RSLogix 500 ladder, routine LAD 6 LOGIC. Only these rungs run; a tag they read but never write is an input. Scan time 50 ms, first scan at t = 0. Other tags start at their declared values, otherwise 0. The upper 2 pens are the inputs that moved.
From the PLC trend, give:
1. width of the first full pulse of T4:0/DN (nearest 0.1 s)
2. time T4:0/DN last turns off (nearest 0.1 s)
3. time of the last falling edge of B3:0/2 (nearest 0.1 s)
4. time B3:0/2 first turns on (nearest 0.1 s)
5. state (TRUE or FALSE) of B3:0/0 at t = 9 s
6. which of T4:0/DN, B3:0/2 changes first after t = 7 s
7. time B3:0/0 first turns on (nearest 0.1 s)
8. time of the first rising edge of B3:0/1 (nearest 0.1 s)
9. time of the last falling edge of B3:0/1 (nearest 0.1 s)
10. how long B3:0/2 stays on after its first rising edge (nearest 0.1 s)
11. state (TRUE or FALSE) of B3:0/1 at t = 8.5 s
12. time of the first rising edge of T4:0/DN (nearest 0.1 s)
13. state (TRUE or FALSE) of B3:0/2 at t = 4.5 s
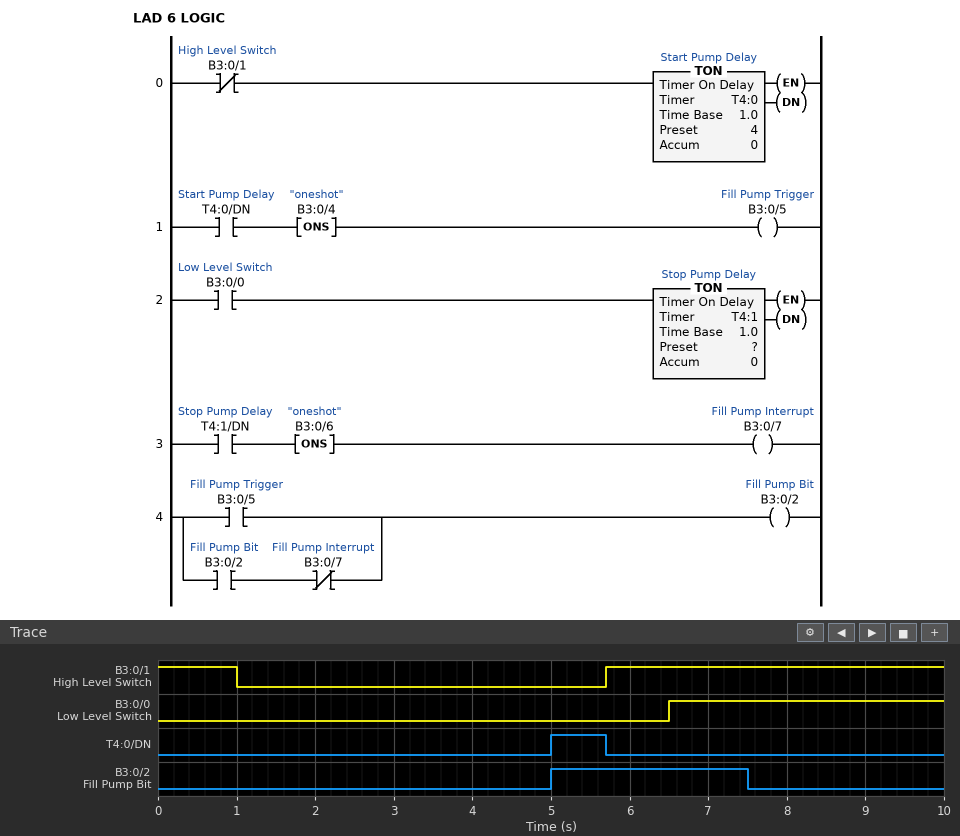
0.7 s
5.7 s
7.5 s
5.0 s
TRUE
B3:0/2
6.5 s
5.7 s
1.0 s
2.5 s
TRUE
5.0 s
FALSE
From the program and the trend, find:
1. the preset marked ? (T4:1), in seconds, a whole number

1 s
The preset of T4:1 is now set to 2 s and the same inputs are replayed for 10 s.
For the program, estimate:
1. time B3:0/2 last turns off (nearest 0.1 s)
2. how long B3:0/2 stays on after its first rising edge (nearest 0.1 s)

8.5 s
3.5 s
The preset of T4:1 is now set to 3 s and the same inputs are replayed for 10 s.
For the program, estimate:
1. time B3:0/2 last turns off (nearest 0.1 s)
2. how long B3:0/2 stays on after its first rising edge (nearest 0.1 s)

9.5 s
4.5 s
